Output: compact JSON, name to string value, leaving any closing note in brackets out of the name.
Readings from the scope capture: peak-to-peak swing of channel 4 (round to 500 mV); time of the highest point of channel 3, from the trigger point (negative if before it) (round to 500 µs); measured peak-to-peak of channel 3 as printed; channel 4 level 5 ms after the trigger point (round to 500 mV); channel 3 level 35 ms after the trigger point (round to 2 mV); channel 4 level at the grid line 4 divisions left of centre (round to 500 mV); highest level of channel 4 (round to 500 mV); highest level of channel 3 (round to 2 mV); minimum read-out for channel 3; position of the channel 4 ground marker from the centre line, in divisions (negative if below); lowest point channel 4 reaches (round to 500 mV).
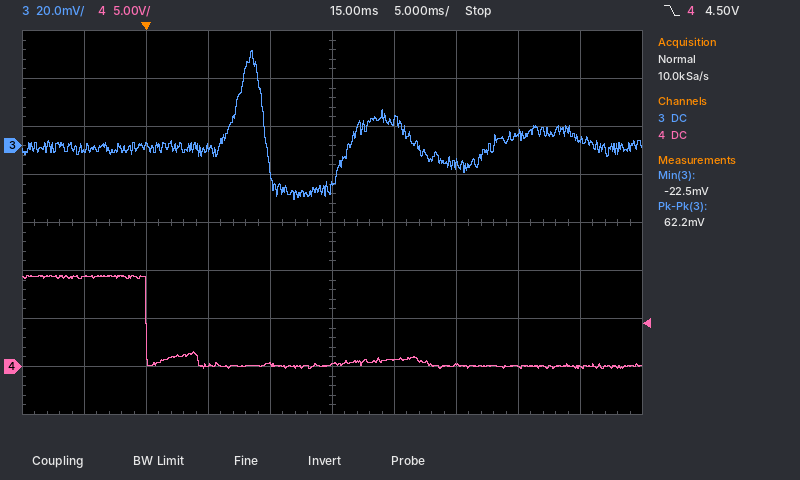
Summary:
{"peak-to-peak swing of channel 4": "9.5 V", "time of the highest point of channel 3, from the trigger point (negative if before it)": "+8.5 ms", "measured peak-to-peak of channel 3 as printed": "62.2 mV", "channel 4 level 5 ms after the trigger point": "0.0 V", "channel 3 level 35 ms after the trigger point": "2 mV", "channel 4 level at the grid line 4 divisions left of centre": "9.5 V", "highest level of channel 4": "9.5 V", "highest level of channel 3": "40 mV", "minimum read-out for channel 3": "-22.5 mV", "position of the channel 4 ground marker from the centre line, in divisions": "-3.0 div", "lowest point channel 4 reaches": "0.0 V"}
